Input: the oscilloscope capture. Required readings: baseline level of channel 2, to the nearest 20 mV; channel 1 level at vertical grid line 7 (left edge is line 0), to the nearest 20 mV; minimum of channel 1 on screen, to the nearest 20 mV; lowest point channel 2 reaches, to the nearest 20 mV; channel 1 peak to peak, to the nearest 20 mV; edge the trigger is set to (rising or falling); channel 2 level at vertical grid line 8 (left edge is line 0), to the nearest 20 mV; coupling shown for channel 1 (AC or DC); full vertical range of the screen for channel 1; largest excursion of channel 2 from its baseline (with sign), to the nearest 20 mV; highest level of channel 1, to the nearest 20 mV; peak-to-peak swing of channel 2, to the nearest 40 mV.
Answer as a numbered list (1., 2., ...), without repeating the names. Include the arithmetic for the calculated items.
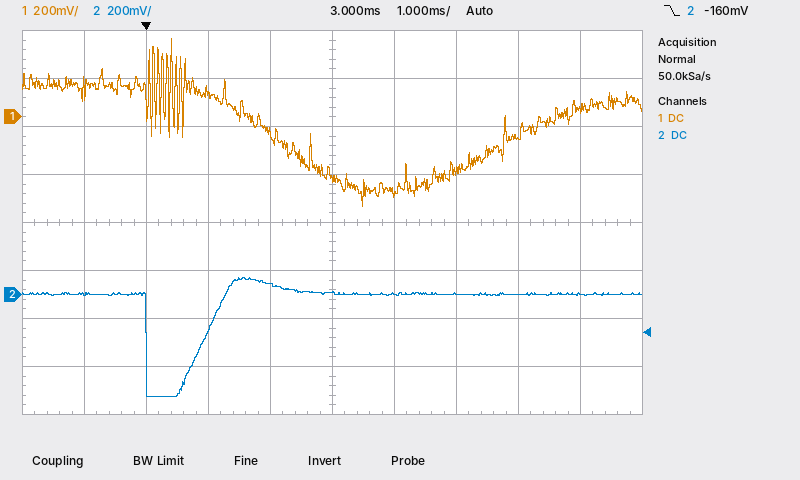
1. 0 mV
2. -220 mV
3. -380 mV
4. -420 mV
5. 320 mV − (-380 mV) = 700 mV
6. falling
7. 0 mV
8. DC
9. 1.6 V
10. -420 mV − (0 mV) = -420 mV
11. 320 mV
12. 480 mV
